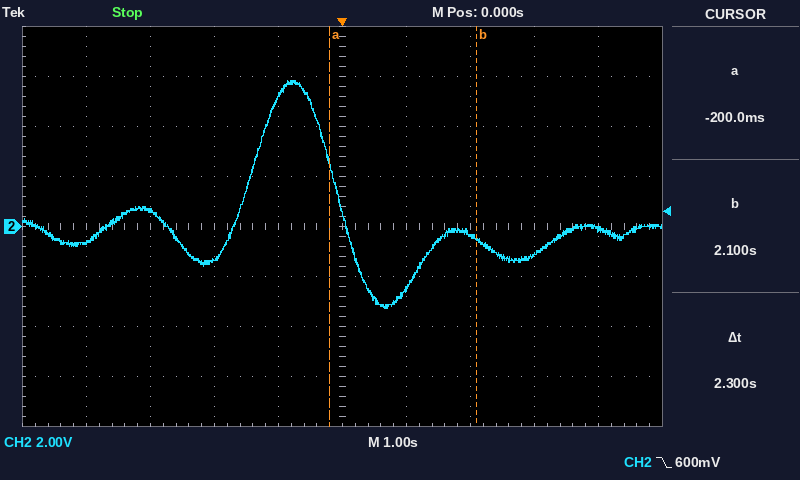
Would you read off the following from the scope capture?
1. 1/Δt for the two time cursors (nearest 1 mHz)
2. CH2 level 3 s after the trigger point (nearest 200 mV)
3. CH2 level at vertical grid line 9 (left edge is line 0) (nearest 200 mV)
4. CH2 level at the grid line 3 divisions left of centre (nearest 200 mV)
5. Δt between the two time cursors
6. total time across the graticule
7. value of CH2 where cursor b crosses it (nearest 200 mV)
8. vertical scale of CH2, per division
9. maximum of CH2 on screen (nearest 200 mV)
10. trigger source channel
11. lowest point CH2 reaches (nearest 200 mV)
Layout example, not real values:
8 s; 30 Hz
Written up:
435 mHz; -1.2 V; -200 mV; 600 mV; 2.3 s; 10 s; -400 mV; 2 V; 5.8 V; CH2; -3.2 V
